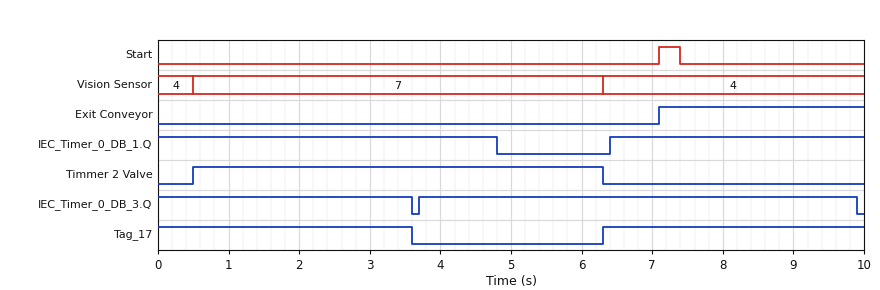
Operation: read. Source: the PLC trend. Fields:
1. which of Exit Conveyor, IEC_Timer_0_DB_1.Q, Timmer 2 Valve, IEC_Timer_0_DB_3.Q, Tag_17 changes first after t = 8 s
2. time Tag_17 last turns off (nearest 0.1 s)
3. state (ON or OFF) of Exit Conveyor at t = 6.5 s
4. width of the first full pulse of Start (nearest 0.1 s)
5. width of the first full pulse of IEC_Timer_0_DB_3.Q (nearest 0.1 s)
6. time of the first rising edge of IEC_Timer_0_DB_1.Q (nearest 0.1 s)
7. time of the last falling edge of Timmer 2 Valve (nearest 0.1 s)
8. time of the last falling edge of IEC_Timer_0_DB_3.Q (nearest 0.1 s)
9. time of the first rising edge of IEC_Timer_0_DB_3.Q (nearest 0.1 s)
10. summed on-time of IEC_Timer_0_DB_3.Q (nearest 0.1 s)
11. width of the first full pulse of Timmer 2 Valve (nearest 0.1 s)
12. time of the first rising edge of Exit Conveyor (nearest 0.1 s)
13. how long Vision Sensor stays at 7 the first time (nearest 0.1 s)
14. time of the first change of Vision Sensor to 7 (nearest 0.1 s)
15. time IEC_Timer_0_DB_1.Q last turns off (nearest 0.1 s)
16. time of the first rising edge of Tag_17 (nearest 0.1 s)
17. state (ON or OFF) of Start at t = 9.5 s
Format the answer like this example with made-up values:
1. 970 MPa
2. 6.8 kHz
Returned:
1. IEC_Timer_0_DB_3.Q
2. 3.6 s
3. OFF
4. 0.3 s
5. 6.2 s
6. 6.4 s
7. 6.3 s
8. 9.9 s
9. 3.7 s
10. 9.8 s
11. 5.8 s
12. 7.1 s
13. 5.8 s
14. 0.5 s
15. 4.8 s
16. 6.3 s
17. OFF
